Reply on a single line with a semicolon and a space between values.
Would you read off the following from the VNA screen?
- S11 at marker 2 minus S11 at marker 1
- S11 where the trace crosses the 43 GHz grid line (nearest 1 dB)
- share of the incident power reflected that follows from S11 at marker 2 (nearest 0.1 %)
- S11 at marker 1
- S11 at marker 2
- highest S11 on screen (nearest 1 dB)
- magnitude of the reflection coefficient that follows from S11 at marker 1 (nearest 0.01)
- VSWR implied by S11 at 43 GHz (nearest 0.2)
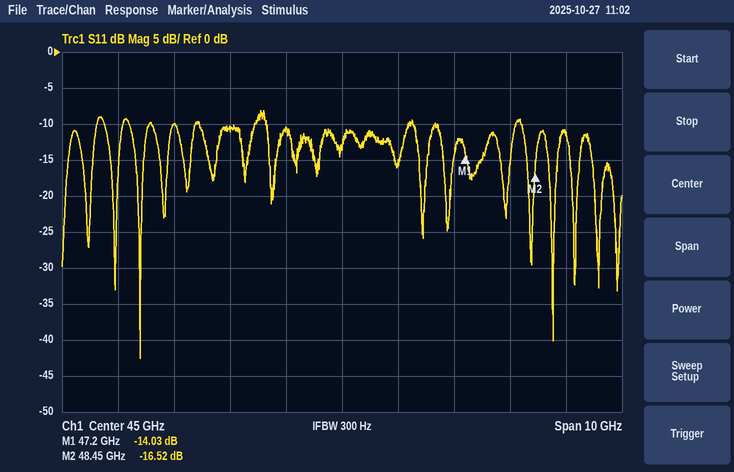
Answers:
-2.49 dB; -11 dB; 2.2 %; -14.03 dB; -16.52 dB; -8 dB; 0.20; 1.8
